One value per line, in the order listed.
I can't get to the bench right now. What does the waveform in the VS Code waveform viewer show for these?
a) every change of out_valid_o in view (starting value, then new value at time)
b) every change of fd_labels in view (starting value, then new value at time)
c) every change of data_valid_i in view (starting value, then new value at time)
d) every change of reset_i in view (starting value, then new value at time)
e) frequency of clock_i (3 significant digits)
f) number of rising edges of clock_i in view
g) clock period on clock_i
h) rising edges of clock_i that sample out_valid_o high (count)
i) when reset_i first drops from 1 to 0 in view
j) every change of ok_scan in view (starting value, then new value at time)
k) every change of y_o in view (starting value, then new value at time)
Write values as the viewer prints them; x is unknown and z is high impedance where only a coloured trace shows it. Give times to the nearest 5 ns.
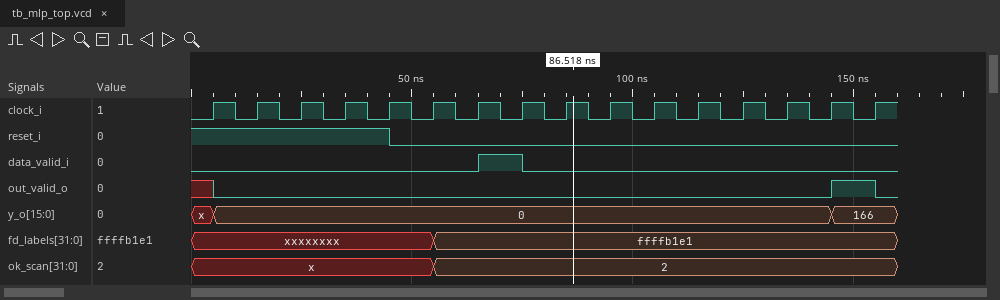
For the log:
x, 0 at 5 ns, 1 at 145 ns, 0 at 155 ns
xxxxxxxx, ffffb1e1 at 55 ns
0, 1 at 65 ns, 0 at 75 ns
1, 0 at 45 ns
100 MHz
16
10 ns
1
45 ns
x, 2 at 55 ns
x, 0 at 5 ns, 166 at 145 ns
